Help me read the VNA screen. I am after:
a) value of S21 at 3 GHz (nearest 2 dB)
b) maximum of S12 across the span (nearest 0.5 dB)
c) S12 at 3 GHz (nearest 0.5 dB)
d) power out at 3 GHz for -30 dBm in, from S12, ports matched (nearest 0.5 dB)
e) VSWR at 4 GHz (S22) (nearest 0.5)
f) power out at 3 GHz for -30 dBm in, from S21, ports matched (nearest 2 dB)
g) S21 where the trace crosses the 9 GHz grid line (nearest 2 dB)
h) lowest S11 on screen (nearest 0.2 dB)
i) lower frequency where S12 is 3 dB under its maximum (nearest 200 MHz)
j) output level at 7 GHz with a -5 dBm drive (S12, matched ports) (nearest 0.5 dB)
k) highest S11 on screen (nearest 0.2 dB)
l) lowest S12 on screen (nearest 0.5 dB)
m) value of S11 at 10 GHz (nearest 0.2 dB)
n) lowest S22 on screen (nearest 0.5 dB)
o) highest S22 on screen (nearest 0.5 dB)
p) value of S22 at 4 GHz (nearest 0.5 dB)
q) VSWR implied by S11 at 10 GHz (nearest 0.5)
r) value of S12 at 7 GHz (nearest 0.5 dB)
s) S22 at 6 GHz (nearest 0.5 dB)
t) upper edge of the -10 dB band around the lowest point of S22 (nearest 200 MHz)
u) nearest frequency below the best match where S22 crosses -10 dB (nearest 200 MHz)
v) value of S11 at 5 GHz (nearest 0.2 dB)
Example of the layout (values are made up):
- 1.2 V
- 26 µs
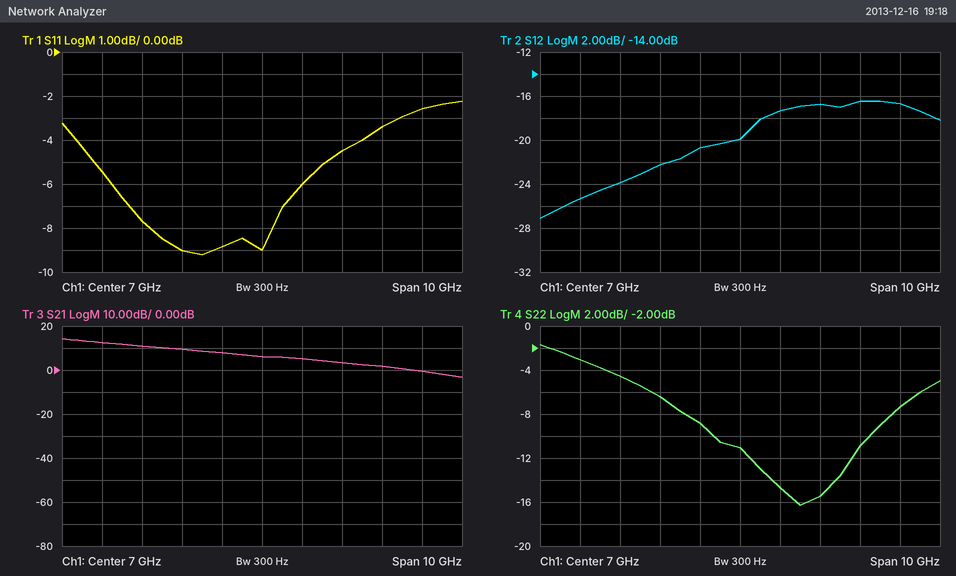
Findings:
- 12 dB
- -16.5 dB
- -25.5 dB
- -55.5 dBm
- 4.0
- -18 dBm
- 4 dB
- -9.2 dB
- 7.2 GHz
- -25.0 dBm
- -2.2 dB
- -27.0 dB
- -3.4 dB
- -16.5 dB
- -1.5 dB
- -4.5 dB
- 5.0
- -20.0 dB
- -9.0 dB
- 10.2 GHz
- 6.4 GHz
- -9.0 dB
